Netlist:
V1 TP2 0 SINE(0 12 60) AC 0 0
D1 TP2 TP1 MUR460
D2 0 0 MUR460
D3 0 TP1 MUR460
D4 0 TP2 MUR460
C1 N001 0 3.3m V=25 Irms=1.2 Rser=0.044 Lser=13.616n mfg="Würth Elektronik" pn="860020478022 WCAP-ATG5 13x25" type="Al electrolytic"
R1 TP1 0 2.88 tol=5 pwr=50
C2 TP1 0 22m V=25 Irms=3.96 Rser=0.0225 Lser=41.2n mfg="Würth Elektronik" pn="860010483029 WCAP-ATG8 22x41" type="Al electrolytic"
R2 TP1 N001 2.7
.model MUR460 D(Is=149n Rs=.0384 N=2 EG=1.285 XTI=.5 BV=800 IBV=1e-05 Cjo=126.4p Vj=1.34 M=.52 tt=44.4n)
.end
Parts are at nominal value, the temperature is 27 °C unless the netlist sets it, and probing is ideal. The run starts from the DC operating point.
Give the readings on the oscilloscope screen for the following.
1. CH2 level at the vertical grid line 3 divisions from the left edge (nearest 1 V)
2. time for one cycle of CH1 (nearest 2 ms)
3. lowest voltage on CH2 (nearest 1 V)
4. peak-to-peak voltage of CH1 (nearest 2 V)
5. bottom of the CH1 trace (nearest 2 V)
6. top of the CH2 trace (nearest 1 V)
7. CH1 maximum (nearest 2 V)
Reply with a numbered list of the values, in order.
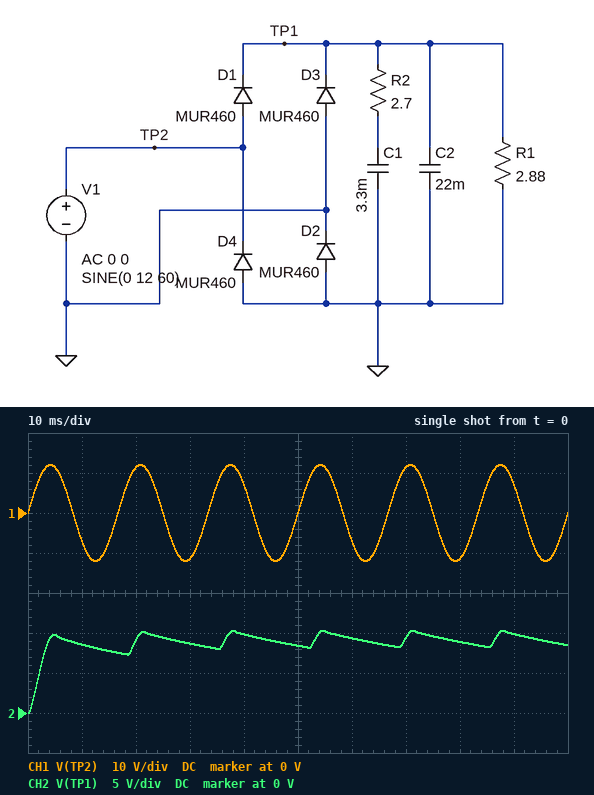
1. 9 V
2. 16 ms
3. 0 V
4. 24 V
5. -12 V
6. 10 V
7. 12 V
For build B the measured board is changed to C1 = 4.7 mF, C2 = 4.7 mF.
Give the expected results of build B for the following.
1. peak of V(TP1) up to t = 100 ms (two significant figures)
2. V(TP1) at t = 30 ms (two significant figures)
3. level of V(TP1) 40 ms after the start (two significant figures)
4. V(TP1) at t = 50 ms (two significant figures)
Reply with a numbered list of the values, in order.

1. 11 V
2. 5.3 V
3. 9.0 V
4. 4.7 V
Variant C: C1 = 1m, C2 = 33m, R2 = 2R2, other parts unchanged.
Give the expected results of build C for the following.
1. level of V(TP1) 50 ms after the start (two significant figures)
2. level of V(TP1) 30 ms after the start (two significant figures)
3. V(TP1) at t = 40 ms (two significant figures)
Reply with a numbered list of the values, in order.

1. 8.8 V
2. 8.9 V
3. 9.7 V
